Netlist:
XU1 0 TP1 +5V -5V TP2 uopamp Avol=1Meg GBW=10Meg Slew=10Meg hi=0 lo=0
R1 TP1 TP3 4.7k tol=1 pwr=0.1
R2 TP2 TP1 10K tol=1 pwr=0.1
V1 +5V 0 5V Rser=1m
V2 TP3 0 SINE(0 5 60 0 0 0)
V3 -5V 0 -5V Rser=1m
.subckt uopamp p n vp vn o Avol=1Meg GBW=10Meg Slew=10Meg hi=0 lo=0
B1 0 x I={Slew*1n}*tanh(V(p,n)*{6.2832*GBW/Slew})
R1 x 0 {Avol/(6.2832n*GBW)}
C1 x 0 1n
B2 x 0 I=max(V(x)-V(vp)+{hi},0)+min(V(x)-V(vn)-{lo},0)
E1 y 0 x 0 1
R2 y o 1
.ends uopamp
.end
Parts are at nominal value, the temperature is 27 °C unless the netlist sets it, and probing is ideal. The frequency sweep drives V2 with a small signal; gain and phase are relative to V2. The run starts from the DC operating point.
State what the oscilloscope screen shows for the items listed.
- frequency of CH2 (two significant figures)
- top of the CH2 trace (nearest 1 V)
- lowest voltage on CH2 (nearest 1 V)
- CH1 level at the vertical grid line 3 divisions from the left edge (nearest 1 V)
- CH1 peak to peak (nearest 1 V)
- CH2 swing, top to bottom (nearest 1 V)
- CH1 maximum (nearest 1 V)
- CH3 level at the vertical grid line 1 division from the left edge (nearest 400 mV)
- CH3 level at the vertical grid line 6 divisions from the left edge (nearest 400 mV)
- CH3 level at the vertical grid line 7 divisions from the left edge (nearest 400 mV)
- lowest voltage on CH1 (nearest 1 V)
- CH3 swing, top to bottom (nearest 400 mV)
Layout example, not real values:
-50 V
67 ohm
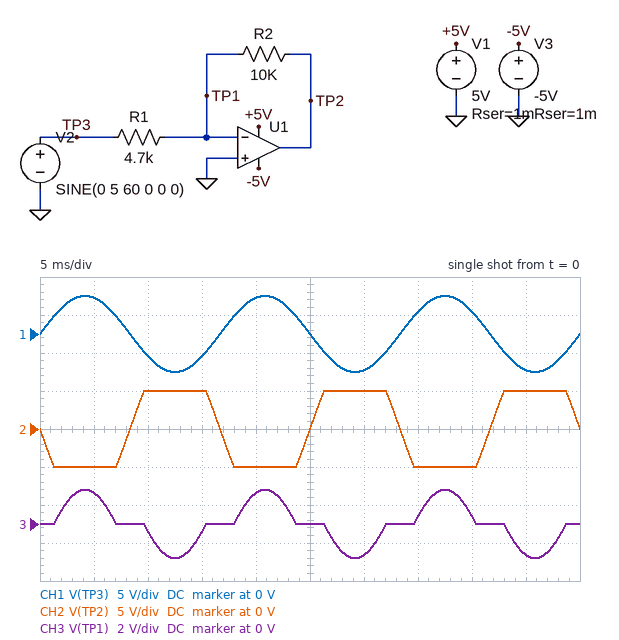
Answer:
60 Hz
5 V
-5 V
-3 V
10 V
10 V
5 V
1.6 V
-1.6 V
400 mV
-5 V
3.6 V
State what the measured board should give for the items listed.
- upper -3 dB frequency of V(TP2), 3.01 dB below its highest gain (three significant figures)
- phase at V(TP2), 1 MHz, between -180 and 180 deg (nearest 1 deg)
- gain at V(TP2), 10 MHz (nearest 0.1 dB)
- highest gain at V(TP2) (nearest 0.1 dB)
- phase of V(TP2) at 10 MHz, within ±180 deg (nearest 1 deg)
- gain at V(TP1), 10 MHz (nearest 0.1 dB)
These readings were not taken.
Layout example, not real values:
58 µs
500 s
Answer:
3.20 MHz
163 deg
-3.8 dB
6.6 dB
108 deg
-3.8 dB
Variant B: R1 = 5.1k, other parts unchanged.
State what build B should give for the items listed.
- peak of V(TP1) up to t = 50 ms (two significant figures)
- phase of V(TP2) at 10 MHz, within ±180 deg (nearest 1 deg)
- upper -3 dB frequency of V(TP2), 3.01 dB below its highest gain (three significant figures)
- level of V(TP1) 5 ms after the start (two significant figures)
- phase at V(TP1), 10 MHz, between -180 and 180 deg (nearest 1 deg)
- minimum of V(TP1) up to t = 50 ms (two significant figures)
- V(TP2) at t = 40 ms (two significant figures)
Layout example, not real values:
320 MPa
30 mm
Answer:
1.6 V
109 deg
3.38 MHz
1.5 V
19 deg
-1.6 V
-5.0 V
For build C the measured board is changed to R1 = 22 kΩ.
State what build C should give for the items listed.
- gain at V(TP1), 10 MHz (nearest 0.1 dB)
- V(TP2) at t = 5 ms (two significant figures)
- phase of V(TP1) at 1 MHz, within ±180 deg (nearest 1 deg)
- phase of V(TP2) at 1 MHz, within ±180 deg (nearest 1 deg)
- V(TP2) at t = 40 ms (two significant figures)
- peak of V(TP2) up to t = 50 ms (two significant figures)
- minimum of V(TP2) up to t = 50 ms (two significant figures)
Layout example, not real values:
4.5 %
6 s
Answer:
-11.8 dB
-2.2 V
82 deg
172 deg
-1.3 V
2.3 V
-2.3 V
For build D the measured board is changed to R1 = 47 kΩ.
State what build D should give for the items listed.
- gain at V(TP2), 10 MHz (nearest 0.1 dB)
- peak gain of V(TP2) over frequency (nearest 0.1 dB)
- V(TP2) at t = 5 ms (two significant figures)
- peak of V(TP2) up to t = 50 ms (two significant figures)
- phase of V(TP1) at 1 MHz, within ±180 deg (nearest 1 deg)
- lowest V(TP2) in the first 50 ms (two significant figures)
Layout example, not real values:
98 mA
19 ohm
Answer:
-17.4 dB
-13.4 dB
-1.0 V
1.1 V
83 deg
-1.1 V
